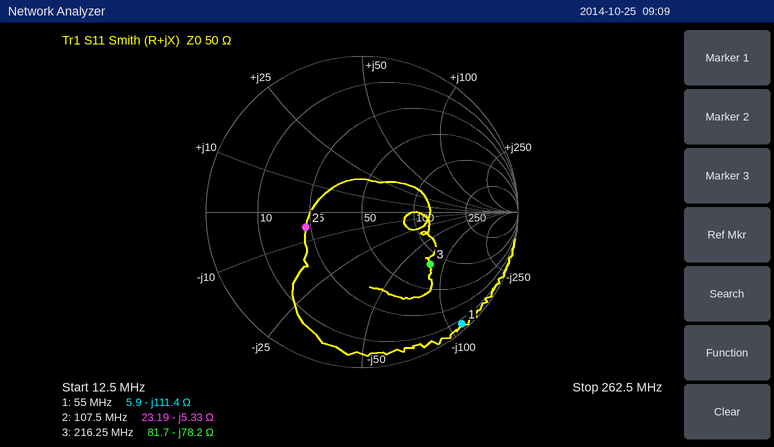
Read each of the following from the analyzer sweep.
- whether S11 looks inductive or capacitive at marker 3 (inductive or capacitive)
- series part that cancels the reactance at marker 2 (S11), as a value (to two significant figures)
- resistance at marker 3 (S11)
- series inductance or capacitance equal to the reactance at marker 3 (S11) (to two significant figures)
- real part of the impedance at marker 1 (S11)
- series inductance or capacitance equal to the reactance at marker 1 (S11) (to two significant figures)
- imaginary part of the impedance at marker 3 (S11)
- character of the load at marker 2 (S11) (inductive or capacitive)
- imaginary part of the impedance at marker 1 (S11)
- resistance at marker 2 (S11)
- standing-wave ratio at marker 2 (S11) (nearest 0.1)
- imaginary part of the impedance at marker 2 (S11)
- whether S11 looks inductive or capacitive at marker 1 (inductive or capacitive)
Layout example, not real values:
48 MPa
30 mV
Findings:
capacitive
7.9 nH
81.7 Ω
9.4 pF
5.9 Ω
26 pF
-78.2 Ω
capacitive
-111.4 Ω
23.19 Ω
2.2
-5.33 Ω
capacitive
